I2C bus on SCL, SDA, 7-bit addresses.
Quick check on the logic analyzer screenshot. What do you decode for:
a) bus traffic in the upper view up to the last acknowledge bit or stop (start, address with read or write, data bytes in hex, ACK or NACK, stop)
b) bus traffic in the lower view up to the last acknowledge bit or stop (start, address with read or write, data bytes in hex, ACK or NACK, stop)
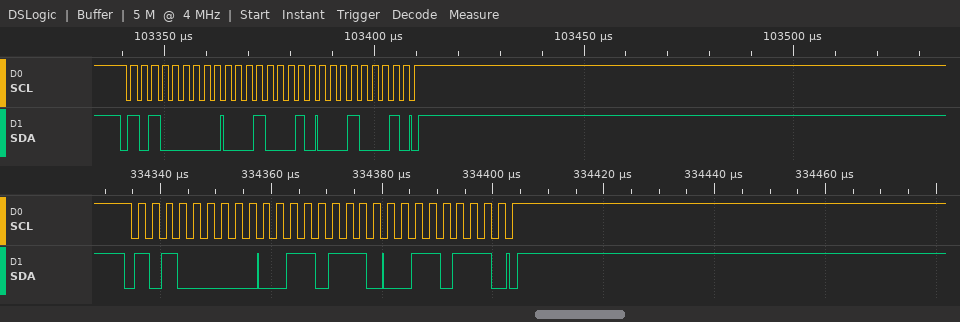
start, address 50 write ACK, 11 ACK, 11 ACK, stop
start, address 50 write ACK, 37 ACK, 37 ACK, stop
